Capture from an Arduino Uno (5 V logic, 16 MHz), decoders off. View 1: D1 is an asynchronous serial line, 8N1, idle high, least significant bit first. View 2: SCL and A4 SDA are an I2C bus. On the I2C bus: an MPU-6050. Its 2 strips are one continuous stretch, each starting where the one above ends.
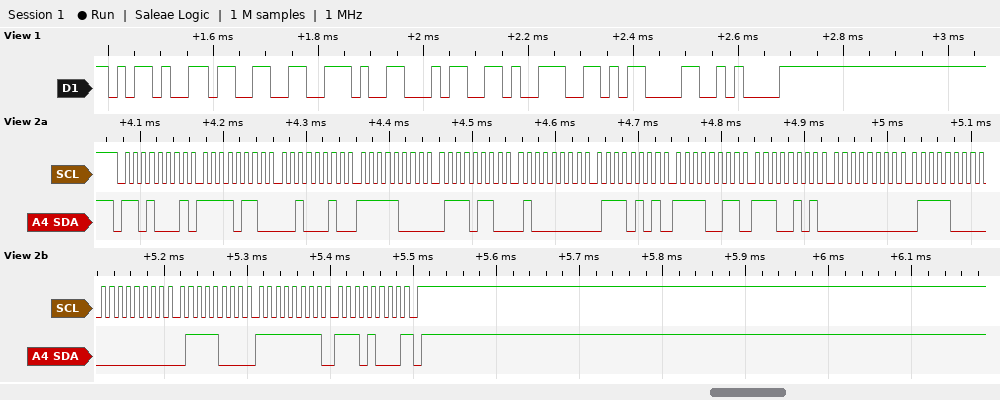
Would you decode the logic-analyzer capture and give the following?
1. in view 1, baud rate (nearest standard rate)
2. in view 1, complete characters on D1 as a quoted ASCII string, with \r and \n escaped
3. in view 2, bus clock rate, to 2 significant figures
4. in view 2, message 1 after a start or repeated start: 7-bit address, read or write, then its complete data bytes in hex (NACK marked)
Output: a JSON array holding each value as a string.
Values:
["57600 baud", "\"-3.49\\r\\n\"", "100 kHz", "0x68 read: F6 22 F8 76 40 75 F3 E5 00 78 00 78 FF E8 NACK"]
